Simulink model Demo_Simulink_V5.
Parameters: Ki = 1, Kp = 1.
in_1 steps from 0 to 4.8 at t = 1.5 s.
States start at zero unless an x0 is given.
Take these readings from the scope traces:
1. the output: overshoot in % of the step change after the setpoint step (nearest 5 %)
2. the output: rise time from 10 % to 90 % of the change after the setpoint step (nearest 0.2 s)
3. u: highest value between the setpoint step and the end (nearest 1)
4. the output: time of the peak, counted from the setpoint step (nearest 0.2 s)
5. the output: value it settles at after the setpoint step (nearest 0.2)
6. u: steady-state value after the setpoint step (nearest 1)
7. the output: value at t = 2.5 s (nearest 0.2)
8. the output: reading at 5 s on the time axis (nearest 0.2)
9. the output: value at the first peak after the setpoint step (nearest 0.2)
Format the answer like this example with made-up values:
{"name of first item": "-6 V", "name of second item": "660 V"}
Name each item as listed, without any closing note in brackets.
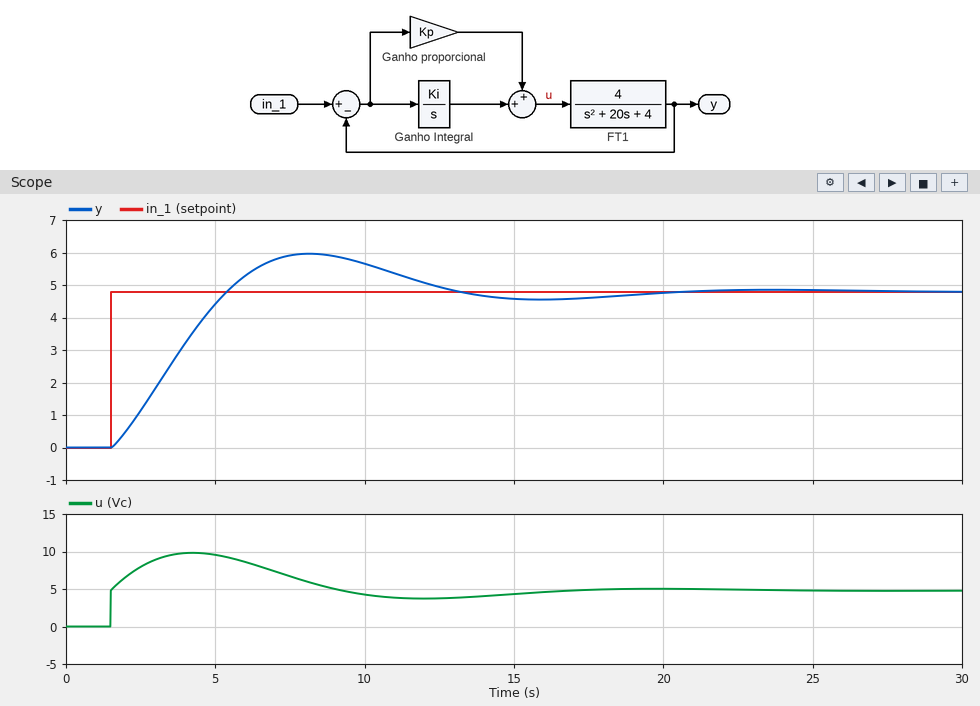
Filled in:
{"the output: overshoot in % of the step change after the setpoint step": "25 %", "the output: rise time from 10 % to 90 % of the change after the setpoint step": "3.0 s", "u: highest value between the setpoint step and the end": "10", "the output: time of the peak, counted from the setpoint step": "6.6 s", "the output: value it settles at after the setpoint step": "4.8", "u: steady-state value after the setpoint step": "5", "the output: value at t = 2.5 s": "1.2", "the output: reading at 5 s on the time axis": "4.4", "the output: value at the first peak after the setpoint step": "6.0"}
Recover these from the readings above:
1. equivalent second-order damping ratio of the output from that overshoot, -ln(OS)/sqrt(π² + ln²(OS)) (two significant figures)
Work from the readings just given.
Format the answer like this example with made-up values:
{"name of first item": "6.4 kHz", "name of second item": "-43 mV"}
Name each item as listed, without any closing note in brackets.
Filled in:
{"equivalent second-order damping ratio of the output from that overshoot, -ln(OS)/sqrt(π² + ln²(OS))": "0.40"}
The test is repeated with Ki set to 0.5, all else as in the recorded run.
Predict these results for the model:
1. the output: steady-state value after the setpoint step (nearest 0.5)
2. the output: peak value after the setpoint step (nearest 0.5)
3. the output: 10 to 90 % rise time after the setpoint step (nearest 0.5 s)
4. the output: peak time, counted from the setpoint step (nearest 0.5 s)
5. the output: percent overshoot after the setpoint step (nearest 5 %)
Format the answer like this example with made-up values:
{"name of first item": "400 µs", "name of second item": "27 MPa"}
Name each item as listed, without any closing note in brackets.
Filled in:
{"the output: steady-state value after the setpoint step": "5.0", "the output: peak value after the setpoint step": "5.5", "the output: 10 to 90 % rise time after the setpoint step": "4.5 s", "the output: peak time, counted from the setpoint step": "10.0 s", "the output: percent overshoot after the setpoint step": "10 %"}
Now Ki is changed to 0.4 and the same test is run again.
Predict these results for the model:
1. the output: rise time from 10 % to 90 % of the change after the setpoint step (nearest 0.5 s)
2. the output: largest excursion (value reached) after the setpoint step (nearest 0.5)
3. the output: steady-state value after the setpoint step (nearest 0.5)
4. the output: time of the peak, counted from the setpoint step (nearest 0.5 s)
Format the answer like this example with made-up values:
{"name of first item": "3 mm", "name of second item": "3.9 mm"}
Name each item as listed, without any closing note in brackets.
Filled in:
{"the output: rise time from 10 % to 90 % of the change after the setpoint step": "5.5 s", "the output: largest excursion (value reached) after the setpoint step": "5.0", "the output: steady-state value after the setpoint step": "5.0", "the output: time of the peak, counted from the setpoint step": "11.5 s"}
